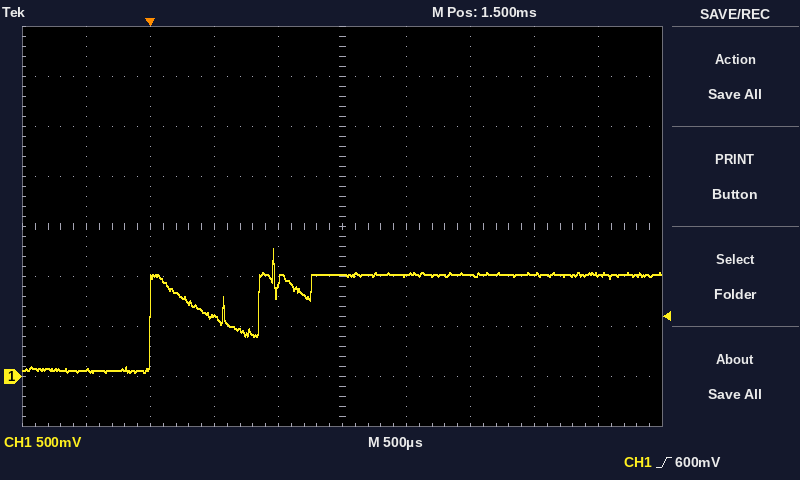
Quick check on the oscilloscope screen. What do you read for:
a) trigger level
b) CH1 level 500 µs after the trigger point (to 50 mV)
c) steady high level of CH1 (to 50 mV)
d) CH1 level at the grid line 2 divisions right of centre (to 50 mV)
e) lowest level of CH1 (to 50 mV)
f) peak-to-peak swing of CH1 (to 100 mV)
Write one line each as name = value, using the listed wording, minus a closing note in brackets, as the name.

trigger level = 600 mV
CH1 level 500 µs after the trigger point = 600 mV
steady high level of CH1 = 1.00 V
CH1 level at the grid line 2 divisions right of centre = 1.00 V
lowest level of CH1 = 50 mV
peak-to-peak swing of CH1 = 1.20 V
